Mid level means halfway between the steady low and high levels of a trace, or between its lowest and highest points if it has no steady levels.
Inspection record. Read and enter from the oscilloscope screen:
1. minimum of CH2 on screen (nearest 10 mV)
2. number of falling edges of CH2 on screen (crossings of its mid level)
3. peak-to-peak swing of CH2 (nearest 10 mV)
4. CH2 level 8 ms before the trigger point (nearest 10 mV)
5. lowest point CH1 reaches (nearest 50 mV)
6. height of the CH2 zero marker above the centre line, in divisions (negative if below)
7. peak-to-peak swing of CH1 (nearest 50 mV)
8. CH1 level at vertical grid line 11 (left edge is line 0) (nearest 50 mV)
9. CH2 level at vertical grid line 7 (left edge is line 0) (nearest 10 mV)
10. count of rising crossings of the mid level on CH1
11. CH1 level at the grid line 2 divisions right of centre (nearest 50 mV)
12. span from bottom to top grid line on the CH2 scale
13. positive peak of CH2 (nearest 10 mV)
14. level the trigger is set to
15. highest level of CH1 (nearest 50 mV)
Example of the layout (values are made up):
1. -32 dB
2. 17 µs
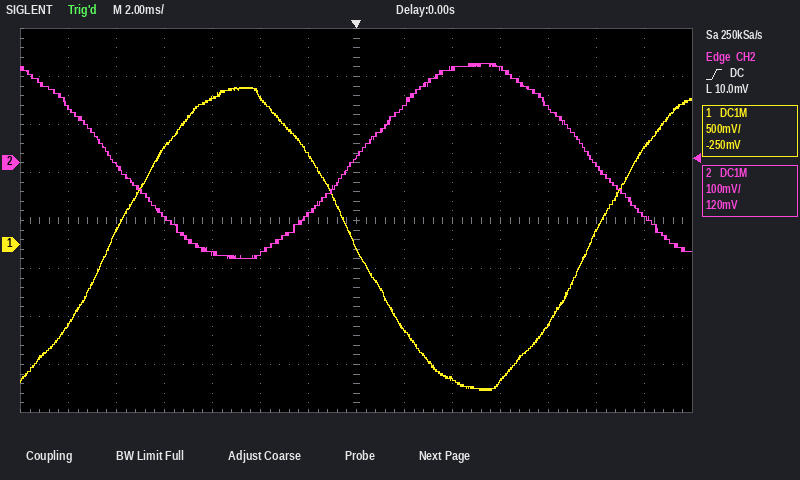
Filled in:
1. -200 mV
2. 2
3. 410 mV
4. -110 mV
5. -1.50 V
6. +1.2 div
7. 3.15 V
8. -850 mV
9. 10 mV
10. 2
11. -1.40 V
12. 800 mV
13. 210 mV
14. 10.0 mV
15. 1.65 V
